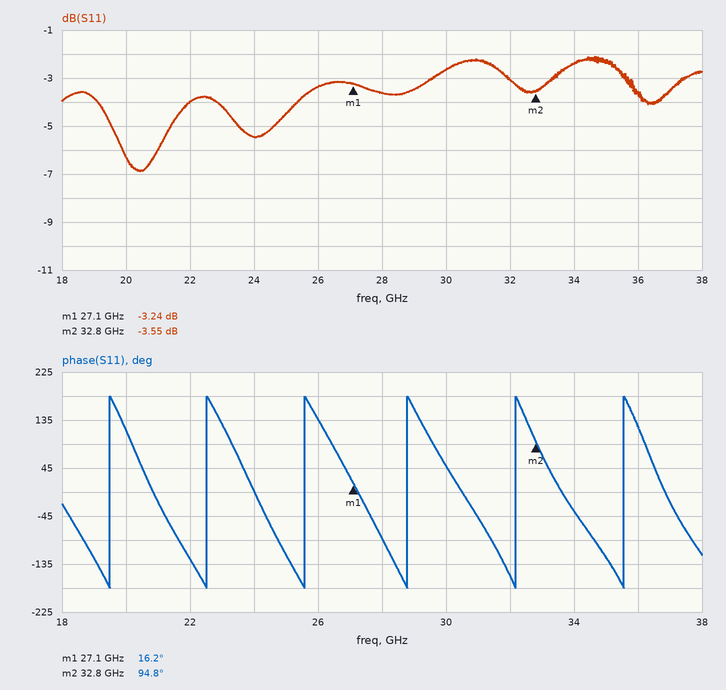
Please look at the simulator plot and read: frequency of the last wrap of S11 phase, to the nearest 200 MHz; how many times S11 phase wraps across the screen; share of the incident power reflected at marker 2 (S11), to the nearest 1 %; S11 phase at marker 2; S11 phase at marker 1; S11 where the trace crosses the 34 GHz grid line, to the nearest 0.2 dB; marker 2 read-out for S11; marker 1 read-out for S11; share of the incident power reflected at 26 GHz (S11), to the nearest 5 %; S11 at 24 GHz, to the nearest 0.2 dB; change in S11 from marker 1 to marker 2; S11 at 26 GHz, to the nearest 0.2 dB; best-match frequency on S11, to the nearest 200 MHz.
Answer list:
35.6 GHz
6
44 %
94.8°
16.2°
-2.4 dB
-3.55 dB
-3.24 dB
45 %
-5.4 dB
-0.31 dB
-3.4 dB
20.4 GHz
